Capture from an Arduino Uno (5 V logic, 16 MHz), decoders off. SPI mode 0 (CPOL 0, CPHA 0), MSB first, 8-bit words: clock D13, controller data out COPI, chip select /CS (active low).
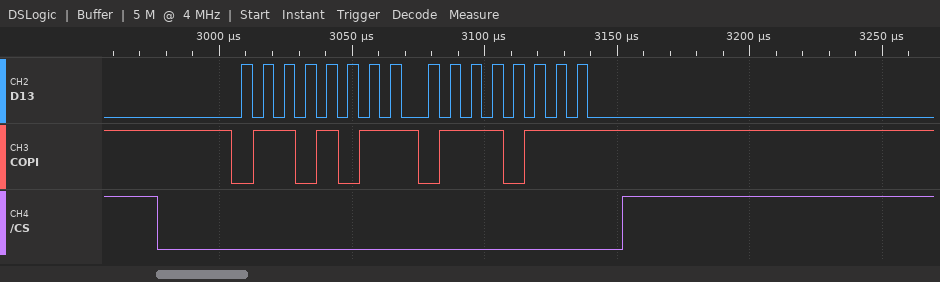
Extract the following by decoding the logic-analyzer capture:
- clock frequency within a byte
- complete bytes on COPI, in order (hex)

125 kHz
6B 77
